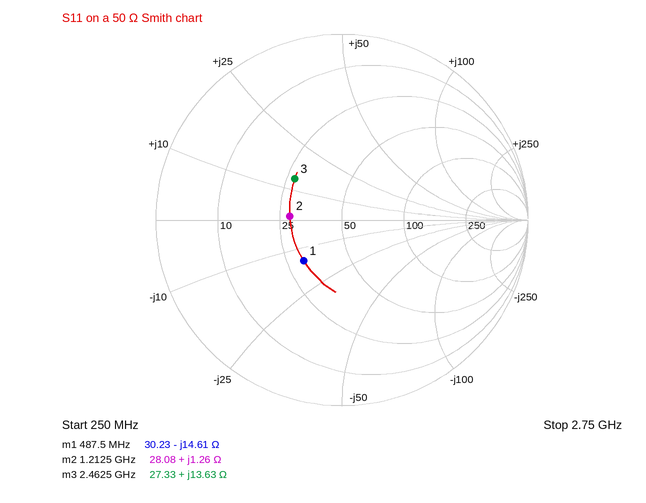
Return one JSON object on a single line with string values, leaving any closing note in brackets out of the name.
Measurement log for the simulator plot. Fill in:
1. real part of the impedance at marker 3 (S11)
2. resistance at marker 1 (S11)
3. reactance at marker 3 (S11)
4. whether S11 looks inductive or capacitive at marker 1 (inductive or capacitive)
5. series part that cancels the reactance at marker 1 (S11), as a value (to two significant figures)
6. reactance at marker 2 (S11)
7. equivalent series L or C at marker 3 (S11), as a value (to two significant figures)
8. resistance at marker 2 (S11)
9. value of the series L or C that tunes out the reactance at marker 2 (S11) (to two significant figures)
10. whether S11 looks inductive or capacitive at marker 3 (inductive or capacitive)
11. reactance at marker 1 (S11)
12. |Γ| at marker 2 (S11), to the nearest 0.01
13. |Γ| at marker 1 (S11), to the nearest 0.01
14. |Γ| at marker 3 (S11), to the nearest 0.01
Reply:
{"real part of the impedance at marker 3": "27.33 Ω", "resistance at marker 1": "30.23 Ω", "reactance at marker 3": "+13.63 Ω", "whether S11 looks inductive or capacitive at marker 1": "capacitive", "series part that cancels the reactance at marker 1 (S11), as a value": "4.8 nH", "reactance at marker 2": "+1.26 Ω", "equivalent series L or C at marker 3 (S11), as a value": "880 pH", "resistance at marker 2": "28.08 Ω", "value of the series L or C that tunes out the reactance at marker 2 (S11)": "100 pF", "whether S11 looks inductive or capacitive at marker 3": "inductive", "reactance at marker 1": "-14.61 Ω", "|Γ| at marker 2 (S11), to the nearest 0.01": "0.28", "|Γ| at marker 1 (S11), to the nearest 0.01": "0.30", "|Γ| at marker 3 (S11), to the nearest 0.01": "0.34"}
